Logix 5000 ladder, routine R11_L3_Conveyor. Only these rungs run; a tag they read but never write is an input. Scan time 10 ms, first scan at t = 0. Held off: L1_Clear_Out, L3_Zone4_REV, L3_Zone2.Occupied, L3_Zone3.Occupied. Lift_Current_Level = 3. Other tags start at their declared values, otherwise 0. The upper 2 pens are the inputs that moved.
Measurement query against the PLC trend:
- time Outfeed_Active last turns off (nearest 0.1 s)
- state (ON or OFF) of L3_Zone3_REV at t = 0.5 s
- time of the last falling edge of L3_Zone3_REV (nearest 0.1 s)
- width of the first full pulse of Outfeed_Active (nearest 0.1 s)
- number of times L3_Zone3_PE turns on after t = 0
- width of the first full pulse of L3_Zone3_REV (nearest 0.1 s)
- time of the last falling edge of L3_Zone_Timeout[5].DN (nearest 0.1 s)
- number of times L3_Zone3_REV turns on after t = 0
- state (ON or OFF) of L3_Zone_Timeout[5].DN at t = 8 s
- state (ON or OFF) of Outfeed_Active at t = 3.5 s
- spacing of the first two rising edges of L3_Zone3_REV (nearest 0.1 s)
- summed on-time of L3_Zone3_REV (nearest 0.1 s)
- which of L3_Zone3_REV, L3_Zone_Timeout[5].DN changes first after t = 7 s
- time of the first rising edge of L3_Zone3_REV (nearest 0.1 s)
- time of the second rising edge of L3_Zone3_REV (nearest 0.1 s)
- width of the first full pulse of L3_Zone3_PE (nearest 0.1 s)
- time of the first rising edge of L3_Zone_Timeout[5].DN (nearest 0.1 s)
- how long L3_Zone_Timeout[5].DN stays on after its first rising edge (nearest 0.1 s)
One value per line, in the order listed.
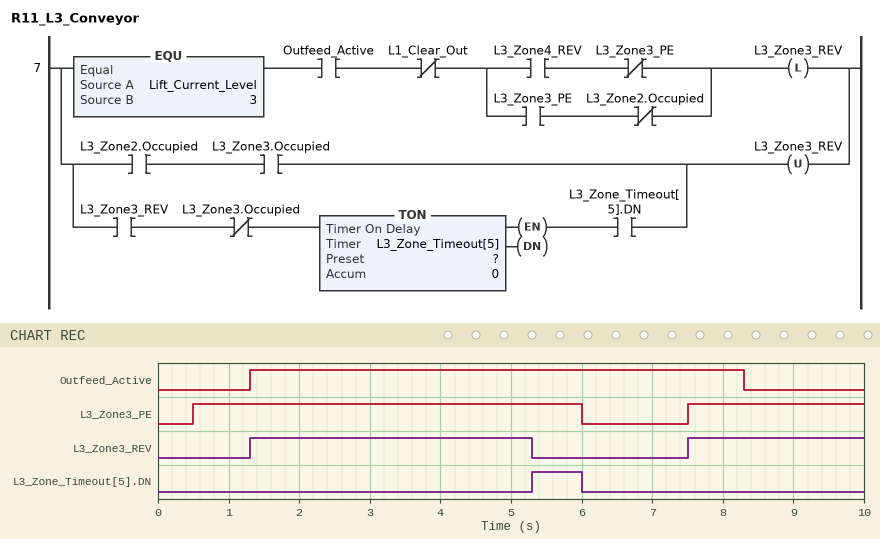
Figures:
8.3 s
OFF
5.3 s
7.0 s
2
4.0 s
6.0 s
2
OFF
ON
6.2 s
6.5 s
L3_Zone3_REV
1.3 s
7.5 s
5.5 s
5.3 s
0.7 s
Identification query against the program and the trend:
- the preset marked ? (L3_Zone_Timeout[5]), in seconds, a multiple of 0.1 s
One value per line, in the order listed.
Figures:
4.0 s
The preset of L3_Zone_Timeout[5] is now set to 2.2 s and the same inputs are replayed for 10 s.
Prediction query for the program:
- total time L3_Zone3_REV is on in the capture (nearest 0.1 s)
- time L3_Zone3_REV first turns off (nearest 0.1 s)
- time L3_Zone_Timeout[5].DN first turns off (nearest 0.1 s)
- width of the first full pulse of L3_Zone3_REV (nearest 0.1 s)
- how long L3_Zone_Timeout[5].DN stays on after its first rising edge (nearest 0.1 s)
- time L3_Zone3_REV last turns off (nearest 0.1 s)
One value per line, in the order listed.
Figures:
4.4 s
3.5 s
6.0 s
2.2 s
2.5 s
9.7 s
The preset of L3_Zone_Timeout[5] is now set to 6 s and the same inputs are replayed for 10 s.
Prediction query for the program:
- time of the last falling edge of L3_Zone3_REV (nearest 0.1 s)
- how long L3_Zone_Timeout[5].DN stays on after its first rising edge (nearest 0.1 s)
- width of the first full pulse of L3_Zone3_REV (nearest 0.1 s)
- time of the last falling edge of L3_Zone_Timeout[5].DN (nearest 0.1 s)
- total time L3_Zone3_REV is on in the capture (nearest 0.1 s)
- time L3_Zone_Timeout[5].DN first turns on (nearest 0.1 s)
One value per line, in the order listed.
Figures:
7.3 s
0.0 s
6.0 s
7.3 s
8.5 s
7.3 s
